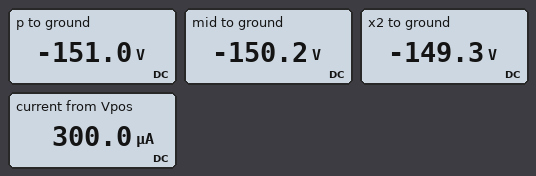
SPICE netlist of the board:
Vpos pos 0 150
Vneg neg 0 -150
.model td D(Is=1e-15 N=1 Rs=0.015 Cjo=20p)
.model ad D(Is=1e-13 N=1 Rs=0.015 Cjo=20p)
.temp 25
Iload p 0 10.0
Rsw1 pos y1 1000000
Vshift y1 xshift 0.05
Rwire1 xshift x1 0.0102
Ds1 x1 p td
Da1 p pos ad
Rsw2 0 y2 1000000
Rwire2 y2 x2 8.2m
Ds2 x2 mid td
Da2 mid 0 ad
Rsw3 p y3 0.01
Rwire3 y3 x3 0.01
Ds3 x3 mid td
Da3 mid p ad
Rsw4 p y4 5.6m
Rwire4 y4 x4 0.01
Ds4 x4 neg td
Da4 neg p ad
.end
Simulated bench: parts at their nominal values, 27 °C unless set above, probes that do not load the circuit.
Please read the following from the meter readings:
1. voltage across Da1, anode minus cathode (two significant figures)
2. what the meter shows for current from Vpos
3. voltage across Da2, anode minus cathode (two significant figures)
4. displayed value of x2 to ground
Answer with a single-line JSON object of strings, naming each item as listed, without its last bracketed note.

{"voltage across Da1, anode minus cathode": "-300 V", "what the meter shows for current from Vpos": "300.0 µA", "voltage across Da2, anode minus cathode": "-150 V", "displayed value of x2 to ground": "-149.3 V"}
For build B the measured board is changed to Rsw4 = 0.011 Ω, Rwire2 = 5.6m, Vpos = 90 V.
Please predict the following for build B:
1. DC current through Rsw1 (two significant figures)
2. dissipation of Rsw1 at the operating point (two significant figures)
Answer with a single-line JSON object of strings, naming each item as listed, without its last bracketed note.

{"DC current through Rsw1": "240 µA", "dissipation of Rsw1 at the operating point": "58 mW"}
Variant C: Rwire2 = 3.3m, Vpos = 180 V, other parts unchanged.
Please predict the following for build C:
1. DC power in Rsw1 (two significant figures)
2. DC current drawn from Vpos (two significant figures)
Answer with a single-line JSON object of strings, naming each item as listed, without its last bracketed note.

{"DC power in Rsw1": "110 mW", "DC current drawn from Vpos": "330 µA"}
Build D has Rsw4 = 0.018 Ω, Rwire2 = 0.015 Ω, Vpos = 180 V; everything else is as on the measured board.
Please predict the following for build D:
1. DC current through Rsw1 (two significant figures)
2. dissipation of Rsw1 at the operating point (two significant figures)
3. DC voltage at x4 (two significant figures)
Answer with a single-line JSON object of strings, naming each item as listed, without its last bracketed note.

{"DC current through Rsw1": "330 µA", "dissipation of Rsw1 at the operating point": "110 mW", "DC voltage at x4": "-150 V"}
